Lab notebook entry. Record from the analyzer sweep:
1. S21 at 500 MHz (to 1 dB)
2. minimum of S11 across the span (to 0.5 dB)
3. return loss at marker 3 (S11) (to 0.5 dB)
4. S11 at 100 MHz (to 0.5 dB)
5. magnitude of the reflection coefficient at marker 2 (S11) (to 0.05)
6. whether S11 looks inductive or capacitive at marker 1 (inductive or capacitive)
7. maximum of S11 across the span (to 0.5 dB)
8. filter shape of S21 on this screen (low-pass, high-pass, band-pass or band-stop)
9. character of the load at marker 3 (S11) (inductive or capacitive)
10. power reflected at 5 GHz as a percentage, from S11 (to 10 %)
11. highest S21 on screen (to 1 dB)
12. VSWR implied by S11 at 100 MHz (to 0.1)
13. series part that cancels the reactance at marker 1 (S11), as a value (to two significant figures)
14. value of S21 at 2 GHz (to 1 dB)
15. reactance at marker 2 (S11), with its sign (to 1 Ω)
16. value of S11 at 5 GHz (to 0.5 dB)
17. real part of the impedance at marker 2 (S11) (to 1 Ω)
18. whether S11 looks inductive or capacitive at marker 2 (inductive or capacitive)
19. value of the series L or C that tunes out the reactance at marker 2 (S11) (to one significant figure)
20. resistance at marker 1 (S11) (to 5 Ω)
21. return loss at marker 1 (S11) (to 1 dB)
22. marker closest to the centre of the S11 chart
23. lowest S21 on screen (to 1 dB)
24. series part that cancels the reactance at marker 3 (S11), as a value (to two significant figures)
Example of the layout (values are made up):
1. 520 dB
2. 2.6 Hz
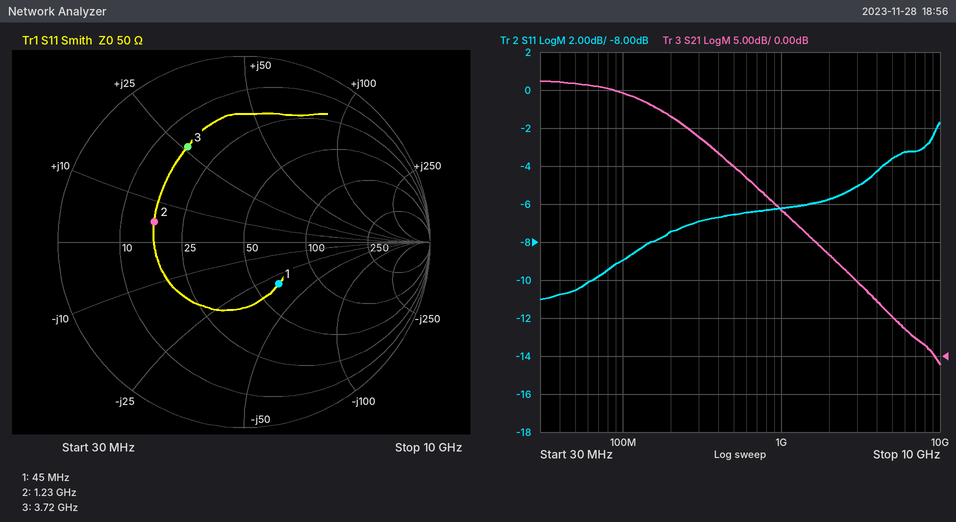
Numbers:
1. 25 dB
2. -11.0 dB
3. 4.5 dB
4. -9.0 dB
5. 0.50
6. capacitive
7. -1.5 dB
8. low-pass
9. inductive
10. 40 %
11. 36 dB
12. 2.1
13. 110 nH
14. 13 dB
15. +5 Ω
16. -3.5 dB
17. 17 Ω
18. inductive
19. 30 pF
20. 65 Ω
21. 11 dB
22. marker 1
23. -1 dB
24. 1.6 pF
